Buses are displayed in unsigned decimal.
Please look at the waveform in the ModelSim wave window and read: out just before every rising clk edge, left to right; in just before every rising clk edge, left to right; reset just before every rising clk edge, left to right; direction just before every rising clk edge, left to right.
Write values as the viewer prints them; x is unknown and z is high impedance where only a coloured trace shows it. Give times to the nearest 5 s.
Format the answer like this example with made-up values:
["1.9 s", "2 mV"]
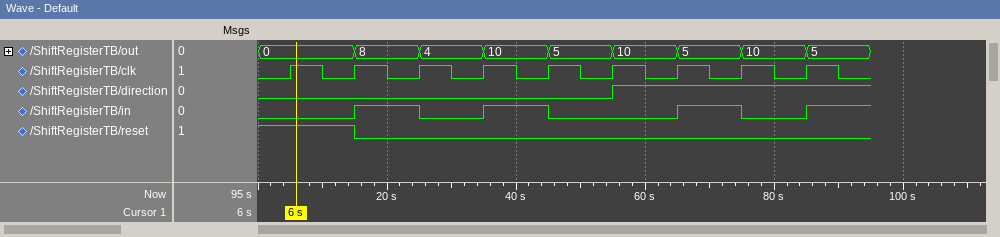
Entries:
["0, 0, 8, 4, 10, 5, 10, 5, 10", "0 0 1 0 1 0 0 1 0", "1 1 0 0 0 0 0 0 0", "0 0 0 0 0 0 1 1 1"]
